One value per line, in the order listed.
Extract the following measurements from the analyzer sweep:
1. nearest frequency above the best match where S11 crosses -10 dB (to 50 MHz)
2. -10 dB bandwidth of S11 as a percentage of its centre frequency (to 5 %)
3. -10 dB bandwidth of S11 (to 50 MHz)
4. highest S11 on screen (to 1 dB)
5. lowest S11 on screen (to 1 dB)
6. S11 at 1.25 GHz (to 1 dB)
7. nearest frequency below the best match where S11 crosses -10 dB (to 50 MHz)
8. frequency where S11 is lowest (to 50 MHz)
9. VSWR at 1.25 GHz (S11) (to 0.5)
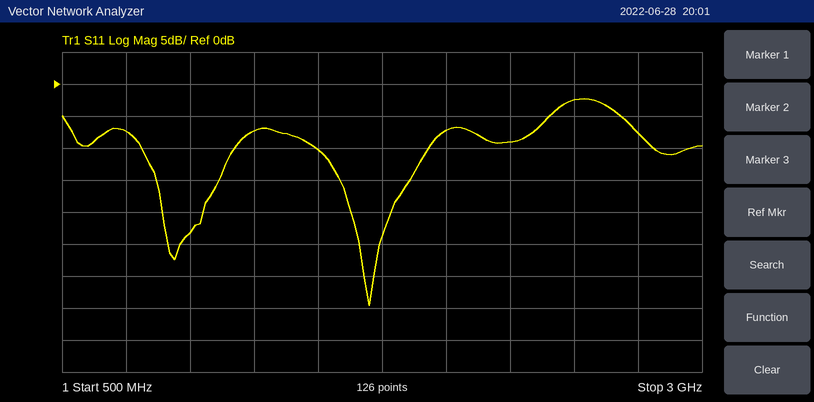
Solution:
1.95 GHz
25 %
450 MHz
-2 dB
-35 dB
-7 dB
1.50 GHz
1.70 GHz
2.5
